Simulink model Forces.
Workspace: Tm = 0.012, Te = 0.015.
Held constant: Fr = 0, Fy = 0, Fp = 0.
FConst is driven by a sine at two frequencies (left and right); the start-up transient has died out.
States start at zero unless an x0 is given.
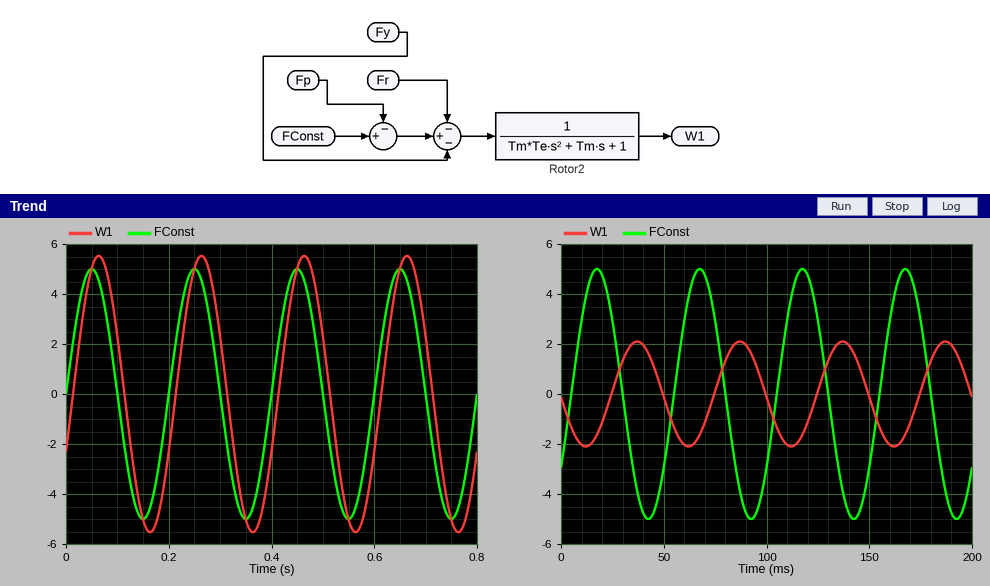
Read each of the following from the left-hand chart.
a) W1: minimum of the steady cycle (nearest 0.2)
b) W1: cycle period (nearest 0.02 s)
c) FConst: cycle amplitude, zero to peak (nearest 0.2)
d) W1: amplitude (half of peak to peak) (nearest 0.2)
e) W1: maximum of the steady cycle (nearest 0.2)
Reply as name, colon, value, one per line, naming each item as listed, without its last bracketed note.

W1: minimum of the steady cycle: -5.6
W1: cycle period: 0.20 s
FConst: cycle amplitude, zero to peak: 5.0
W1: amplitude (half of peak to peak): 5.6
W1: maximum of the steady cycle: 5.6
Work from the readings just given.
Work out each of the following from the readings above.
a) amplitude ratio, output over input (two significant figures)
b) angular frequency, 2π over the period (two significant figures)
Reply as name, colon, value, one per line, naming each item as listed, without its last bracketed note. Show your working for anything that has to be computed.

amplitude ratio, output over input: 5.6 / 5 = 1.1
angular frequency, 2π over the period: 2π / 0.2 = 31 rad/s
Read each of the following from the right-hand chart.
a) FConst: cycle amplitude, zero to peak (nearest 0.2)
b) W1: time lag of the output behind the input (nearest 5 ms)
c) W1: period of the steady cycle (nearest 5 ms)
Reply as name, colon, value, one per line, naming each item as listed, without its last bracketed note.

FConst: cycle amplitude, zero to peak: 5.0
W1: time lag of the output behind the input: 20 ms
W1: period of the steady cycle: 50 ms
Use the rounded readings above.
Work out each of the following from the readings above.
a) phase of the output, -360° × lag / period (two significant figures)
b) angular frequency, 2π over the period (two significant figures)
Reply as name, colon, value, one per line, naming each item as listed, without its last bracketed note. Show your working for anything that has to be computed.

phase of the output, -360° × lag / period: -360 × 20 / 50 = -140°
angular frequency, 2π over the period: 2π / 50 = 0.13 rad/ms
